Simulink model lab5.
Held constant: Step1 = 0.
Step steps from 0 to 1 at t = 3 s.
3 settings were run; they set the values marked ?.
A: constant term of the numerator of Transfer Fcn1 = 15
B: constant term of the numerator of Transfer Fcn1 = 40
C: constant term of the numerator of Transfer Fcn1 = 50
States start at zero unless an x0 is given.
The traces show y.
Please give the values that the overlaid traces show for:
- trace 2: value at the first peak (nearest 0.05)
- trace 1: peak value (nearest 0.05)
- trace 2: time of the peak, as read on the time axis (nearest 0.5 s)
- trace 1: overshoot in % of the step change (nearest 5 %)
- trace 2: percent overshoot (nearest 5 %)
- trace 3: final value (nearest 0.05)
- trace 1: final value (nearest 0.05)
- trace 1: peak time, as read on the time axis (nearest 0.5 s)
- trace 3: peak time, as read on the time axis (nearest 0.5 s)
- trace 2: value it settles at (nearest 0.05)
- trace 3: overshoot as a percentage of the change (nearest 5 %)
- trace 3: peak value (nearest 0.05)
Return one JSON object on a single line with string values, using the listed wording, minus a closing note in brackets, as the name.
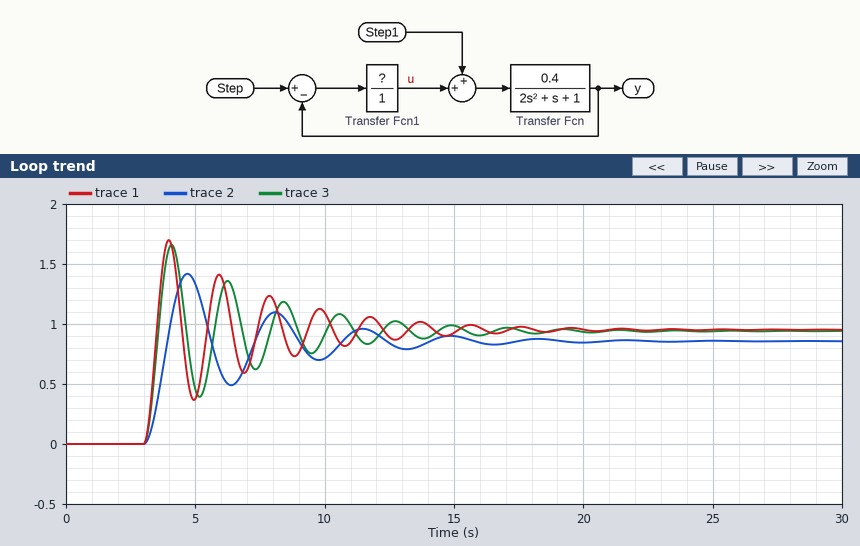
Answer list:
{"trace 2: value at the first peak": "1.40", "trace 1: peak value": "1.70", "trace 2: time of the peak, as read on the time axis": "4.5 s", "trace 1: overshoot in % of the step change": "80 %", "trace 2: percent overshoot": "65 %", "trace 3: final value": "0.95", "trace 1: final value": "0.95", "trace 1: peak time, as read on the time axis": "4.0 s", "trace 3: peak time, as read on the time axis": "4.0 s", "trace 2: value it settles at": "0.85", "trace 3: overshoot as a percentage of the change": "75 %", "trace 3: peak value": "1.65"}
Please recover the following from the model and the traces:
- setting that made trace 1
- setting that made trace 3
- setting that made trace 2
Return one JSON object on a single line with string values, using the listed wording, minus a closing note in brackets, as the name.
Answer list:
{"setting that made trace 1": "C", "setting that made trace 3": "B", "setting that made trace 2": "A"}
